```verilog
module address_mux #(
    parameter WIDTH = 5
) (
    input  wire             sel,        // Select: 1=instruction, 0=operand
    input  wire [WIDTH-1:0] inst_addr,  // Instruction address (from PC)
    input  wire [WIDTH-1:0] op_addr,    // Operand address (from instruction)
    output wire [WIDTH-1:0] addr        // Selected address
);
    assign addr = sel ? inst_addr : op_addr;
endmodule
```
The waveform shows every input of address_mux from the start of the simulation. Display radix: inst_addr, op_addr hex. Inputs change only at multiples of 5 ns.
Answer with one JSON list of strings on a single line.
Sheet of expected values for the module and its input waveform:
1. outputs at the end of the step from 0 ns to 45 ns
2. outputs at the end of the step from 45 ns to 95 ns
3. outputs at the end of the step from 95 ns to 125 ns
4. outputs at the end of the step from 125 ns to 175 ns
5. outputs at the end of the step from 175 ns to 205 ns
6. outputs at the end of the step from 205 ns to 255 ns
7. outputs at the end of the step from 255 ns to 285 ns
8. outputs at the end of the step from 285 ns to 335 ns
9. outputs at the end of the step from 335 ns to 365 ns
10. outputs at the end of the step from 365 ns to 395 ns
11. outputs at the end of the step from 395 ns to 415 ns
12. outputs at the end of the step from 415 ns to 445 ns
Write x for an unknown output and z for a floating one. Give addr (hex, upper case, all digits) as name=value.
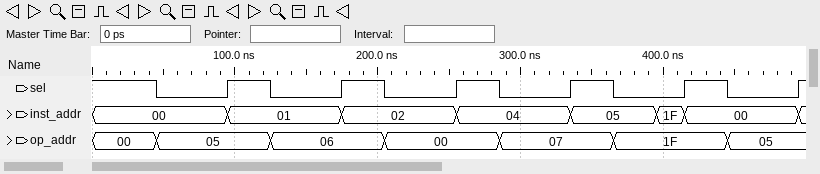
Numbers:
["addr=00", "addr=05", "addr=01", "addr=06", "addr=02", "addr=00", "addr=04", "addr=07", "addr=05", "addr=1F", "addr=1F", "addr=00"]
